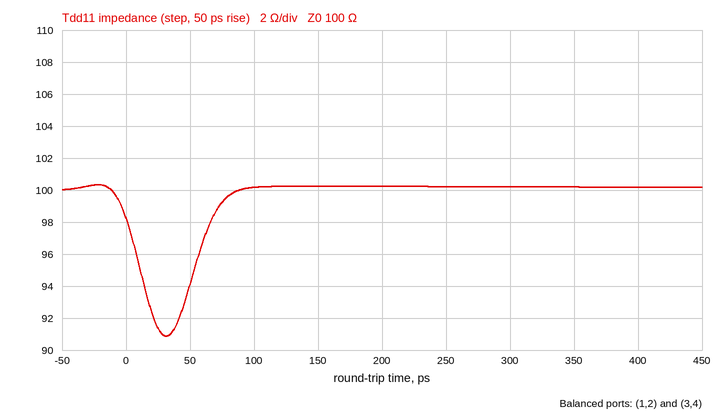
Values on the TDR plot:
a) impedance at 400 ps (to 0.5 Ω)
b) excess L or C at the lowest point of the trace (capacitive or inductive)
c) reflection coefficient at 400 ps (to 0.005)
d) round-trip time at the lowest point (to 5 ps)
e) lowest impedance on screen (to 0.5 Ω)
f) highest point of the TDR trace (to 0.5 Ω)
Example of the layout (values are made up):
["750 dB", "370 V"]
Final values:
["100.0 Ω", "capacitive", "0.000", "30 ps", "91.0 Ω", "100.5 Ω"]
